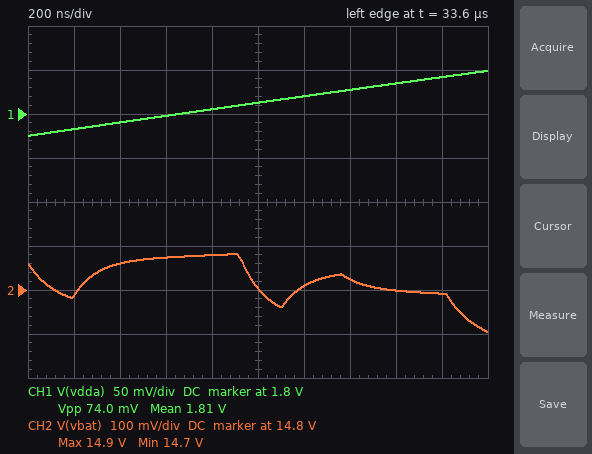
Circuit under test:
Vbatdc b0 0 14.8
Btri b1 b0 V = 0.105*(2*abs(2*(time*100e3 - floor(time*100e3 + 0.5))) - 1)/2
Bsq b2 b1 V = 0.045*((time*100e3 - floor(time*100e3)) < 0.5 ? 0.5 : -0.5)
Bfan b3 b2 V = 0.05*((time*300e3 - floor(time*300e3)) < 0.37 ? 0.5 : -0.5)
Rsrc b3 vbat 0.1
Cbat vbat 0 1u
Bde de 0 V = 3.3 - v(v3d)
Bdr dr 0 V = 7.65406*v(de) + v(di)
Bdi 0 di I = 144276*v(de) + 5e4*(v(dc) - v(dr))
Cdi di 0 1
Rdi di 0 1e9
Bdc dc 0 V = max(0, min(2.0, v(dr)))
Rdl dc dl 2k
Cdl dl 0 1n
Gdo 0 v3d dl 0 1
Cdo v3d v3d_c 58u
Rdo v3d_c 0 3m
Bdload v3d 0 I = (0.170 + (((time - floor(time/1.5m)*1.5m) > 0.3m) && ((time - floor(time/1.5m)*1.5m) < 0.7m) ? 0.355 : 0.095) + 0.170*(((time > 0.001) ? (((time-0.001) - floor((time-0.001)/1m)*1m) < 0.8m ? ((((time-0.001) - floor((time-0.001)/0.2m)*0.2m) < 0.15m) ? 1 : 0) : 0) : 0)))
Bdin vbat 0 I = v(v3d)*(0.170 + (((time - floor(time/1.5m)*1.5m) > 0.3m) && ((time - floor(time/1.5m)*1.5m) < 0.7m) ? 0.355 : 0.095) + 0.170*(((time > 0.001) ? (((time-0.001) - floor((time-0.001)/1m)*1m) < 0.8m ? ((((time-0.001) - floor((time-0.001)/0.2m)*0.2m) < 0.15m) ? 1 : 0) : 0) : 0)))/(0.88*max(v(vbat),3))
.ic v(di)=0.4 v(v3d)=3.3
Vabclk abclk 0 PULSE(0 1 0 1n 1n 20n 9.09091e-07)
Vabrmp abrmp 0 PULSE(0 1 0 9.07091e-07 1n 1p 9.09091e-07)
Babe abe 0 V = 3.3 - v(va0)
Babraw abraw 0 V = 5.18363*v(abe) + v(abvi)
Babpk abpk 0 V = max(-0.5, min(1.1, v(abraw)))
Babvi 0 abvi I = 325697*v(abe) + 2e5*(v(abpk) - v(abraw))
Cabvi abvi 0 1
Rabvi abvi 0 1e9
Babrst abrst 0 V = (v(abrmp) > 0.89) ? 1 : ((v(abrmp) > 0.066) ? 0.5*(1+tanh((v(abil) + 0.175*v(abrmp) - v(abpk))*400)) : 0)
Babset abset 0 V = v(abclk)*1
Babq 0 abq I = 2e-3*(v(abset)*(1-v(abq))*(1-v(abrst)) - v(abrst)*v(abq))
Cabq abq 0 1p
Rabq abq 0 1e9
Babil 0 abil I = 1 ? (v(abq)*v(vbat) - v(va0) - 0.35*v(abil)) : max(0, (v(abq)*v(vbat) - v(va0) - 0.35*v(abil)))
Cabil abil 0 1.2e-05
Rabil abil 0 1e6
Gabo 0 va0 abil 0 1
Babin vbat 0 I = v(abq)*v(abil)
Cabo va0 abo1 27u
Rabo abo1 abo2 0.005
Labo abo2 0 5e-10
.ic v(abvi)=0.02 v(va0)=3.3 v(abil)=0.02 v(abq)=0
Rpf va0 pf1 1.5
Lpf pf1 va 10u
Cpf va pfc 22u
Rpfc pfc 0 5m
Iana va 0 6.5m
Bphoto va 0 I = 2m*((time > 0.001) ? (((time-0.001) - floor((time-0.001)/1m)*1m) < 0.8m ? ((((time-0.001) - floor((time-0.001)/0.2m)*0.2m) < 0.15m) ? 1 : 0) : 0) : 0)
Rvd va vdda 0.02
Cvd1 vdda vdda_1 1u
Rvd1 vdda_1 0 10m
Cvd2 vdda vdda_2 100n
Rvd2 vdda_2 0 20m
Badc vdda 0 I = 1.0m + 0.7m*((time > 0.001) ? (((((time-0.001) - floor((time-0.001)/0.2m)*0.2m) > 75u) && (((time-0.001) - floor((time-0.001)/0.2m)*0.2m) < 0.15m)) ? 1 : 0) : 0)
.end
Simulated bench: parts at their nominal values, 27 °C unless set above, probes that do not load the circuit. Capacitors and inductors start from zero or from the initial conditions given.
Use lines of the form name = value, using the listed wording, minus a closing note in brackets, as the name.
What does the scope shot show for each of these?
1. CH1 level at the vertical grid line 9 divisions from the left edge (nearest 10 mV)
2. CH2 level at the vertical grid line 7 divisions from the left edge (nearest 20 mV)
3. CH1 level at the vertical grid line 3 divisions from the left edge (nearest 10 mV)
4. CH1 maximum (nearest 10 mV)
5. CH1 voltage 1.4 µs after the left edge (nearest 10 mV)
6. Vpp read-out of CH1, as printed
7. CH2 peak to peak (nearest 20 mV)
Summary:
CH1 level at the vertical grid line 9 divisions from the left edge = 1.84 V
CH2 level at the vertical grid line 7 divisions from the left edge = 14.82 V
CH1 level at the vertical grid line 3 divisions from the left edge = 1.80 V
CH1 maximum = 1.85 V
CH1 voltage 1.4 µs after the left edge = 1.83 V
Vpp read-out of CH1, as printed = 74.0 mV
CH2 peak to peak = 180 mV
